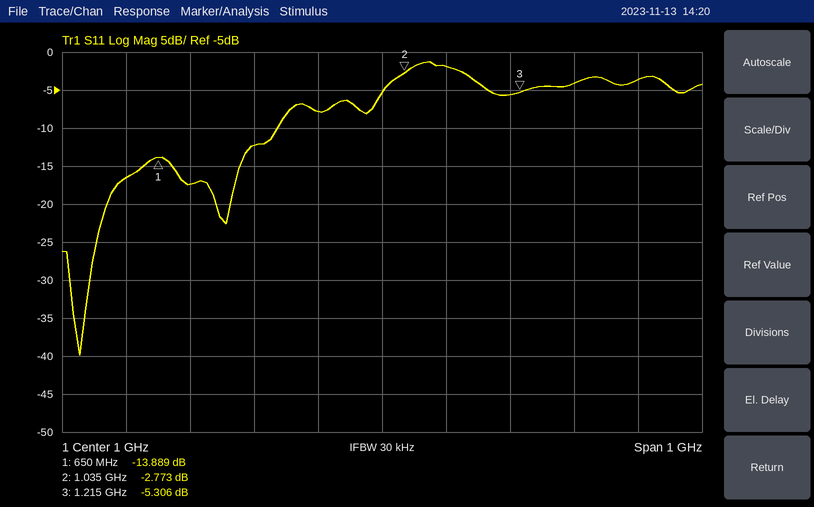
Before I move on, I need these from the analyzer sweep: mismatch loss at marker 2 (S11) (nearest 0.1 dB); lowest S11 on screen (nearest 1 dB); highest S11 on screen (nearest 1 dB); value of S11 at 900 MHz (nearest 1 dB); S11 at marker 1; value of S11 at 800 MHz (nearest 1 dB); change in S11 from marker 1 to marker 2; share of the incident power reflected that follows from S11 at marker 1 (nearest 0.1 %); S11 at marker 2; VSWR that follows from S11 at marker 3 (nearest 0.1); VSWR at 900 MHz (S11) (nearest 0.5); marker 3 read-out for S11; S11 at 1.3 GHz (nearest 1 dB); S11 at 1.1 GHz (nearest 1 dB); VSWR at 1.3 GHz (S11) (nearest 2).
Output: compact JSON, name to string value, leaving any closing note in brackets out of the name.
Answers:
{"mismatch loss at marker 2 (S11)": "3.3 dB", "lowest S11 on screen": "-40 dB", "highest S11 on screen": "-1 dB", "value of S11 at 900 MHz": "-8 dB", "S11 at marker 1": "-13.889 dB", "value of S11 at 800 MHz": "-12 dB", "change in S11 from marker 1 to marker 2": "11.116 dB", "share of the incident power reflected that follows from S11 at marker 1": "4.1 %", "S11 at marker 2": "-2.773 dB", "VSWR that follows from S11 at marker 3": "3.4", "VSWR at 900 MHz (S11)": "2.5", "marker 3 read-out for S11": "-5.306 dB", "S11 at 1.3 GHz": "-4 dB", "S11 at 1.1 GHz": "-2 dB", "VSWR at 1.3 GHz (S11)": "4"}
